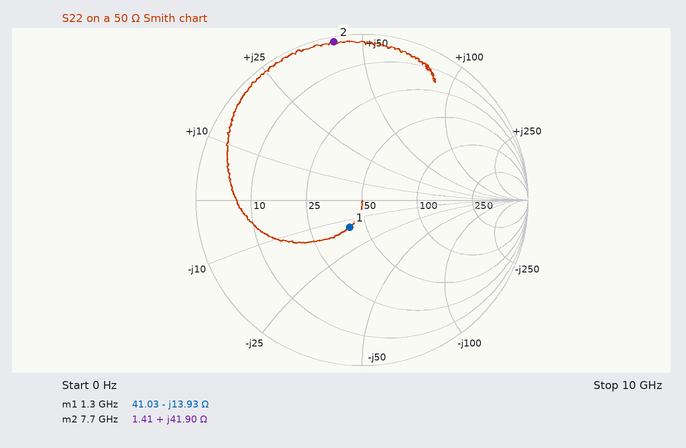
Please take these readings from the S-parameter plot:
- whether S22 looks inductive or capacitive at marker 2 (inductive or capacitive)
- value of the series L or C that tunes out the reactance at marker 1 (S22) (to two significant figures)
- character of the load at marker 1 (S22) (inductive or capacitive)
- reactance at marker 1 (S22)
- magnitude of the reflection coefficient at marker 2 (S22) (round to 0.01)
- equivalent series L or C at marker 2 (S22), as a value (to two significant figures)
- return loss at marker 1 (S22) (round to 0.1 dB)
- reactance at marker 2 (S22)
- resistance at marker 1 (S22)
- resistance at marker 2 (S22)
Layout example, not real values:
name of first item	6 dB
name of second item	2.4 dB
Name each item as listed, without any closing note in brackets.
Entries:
whether S22 looks inductive or capacitive at marker 2	inductive
value of the series L or C that tunes out the reactance at marker 1 (S22)	1.7 nH
character of the load at marker 1 (S22)	capacitive
reactance at marker 1	-13.93 Ω
magnitude of the reflection coefficient at marker 2 (S22)	0.97
equivalent series L or C at marker 2 (S22), as a value	870 pH
return loss at marker 1 (S22)	14.9 dB
reactance at marker 2	+41.90 Ω
resistance at marker 1	41.03 Ω
resistance at marker 2	1.41 Ω
